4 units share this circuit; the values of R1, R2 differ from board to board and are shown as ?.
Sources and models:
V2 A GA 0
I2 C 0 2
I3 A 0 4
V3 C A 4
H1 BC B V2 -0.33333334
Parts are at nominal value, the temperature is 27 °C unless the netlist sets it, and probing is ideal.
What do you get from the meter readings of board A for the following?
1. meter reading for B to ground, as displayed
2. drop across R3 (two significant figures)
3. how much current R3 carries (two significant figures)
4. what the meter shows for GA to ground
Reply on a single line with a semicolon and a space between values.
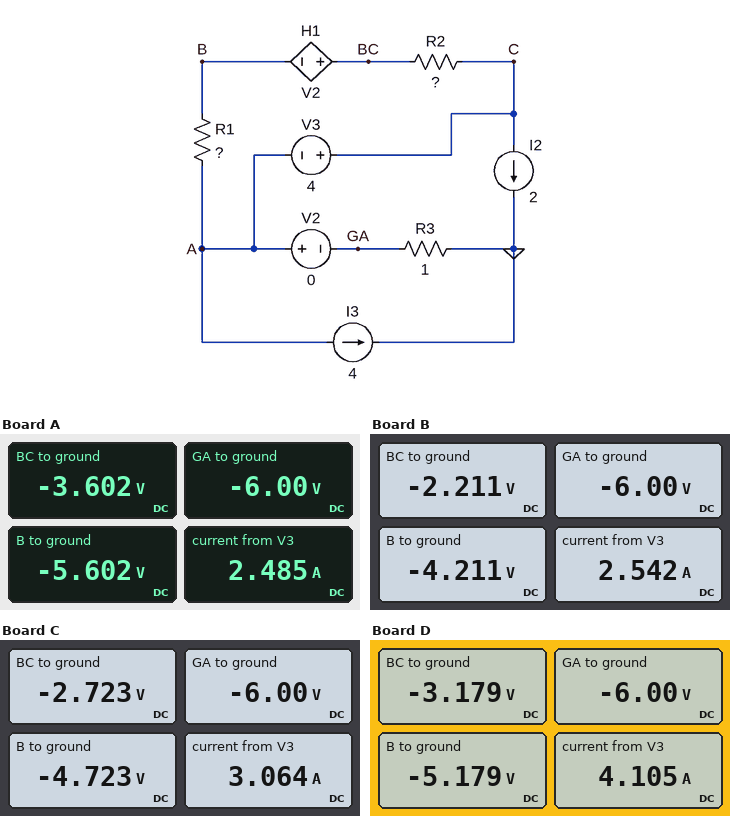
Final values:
-5.602 V; 6.0 V; 6.0 A; -6.00 V
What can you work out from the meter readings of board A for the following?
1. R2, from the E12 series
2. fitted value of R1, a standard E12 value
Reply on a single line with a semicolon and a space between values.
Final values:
3.3 Ω; 0.82 Ω
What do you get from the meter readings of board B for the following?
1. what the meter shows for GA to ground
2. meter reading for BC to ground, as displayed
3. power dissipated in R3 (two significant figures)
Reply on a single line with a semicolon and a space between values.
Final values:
-6.00 V; -2.211 V; 36 W
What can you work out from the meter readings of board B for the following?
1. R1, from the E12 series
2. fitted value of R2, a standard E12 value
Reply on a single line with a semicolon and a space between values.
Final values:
3.3 Ω; 0.39 Ω
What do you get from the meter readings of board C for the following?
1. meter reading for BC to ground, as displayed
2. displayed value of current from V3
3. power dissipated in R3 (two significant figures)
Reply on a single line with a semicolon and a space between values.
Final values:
-2.723 V; 3.064 A; 36 W
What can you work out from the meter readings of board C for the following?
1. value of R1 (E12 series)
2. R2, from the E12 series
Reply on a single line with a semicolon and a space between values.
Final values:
1.2 Ω; 0.68 Ω
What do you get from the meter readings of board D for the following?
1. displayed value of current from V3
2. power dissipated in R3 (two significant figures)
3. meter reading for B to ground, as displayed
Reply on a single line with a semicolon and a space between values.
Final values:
4.105 A; 36 W; -5.179 V
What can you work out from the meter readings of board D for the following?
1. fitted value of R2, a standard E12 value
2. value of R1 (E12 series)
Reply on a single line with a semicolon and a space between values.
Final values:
0.56 Ω; 0.39 Ω
